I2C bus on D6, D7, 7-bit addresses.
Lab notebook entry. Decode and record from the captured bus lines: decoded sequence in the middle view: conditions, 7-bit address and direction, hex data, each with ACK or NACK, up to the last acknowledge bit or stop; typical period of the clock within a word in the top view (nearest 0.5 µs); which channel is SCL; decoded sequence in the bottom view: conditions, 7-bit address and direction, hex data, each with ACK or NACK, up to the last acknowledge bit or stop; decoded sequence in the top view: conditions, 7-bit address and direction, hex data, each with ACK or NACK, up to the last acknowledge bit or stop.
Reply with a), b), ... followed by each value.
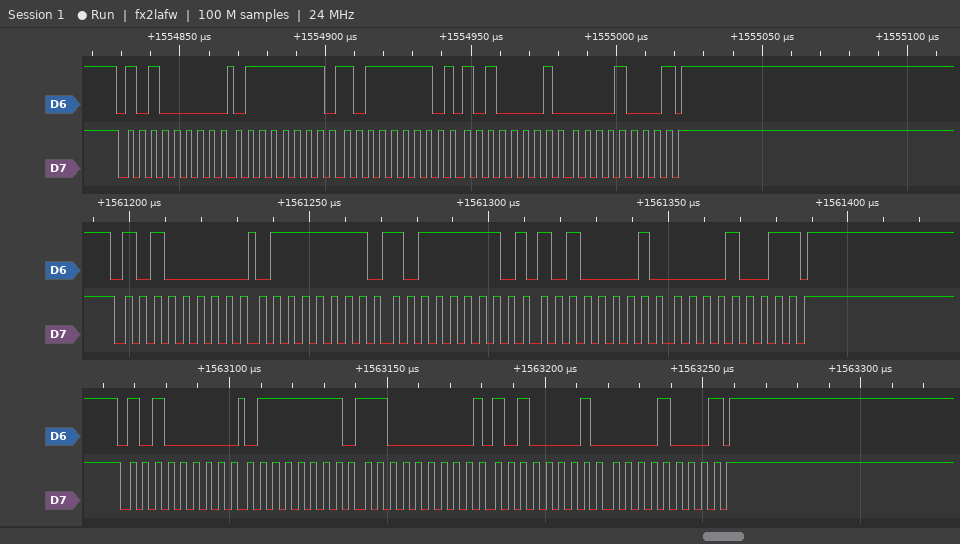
a) start, address 50 write ACK, 7F ACK, BF ACK, repeated start, address 50 read ACK, 09 NACK, stop
b) 4 µs
c) D7
d) start, address 50 write ACK, 7F ACK, C0 ACK, repeated start, address 50 read ACK, 08 NACK, stop
e) start, address 50 write ACK, 7F ACK, BF ACK, repeated start, address 50 read ACK, 08 NACK, stop
